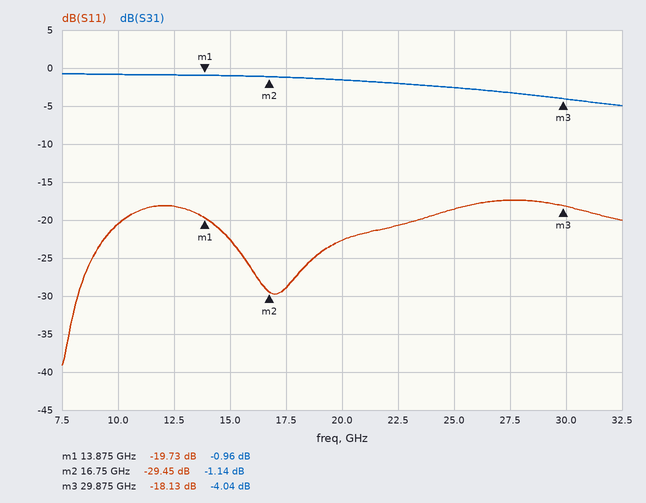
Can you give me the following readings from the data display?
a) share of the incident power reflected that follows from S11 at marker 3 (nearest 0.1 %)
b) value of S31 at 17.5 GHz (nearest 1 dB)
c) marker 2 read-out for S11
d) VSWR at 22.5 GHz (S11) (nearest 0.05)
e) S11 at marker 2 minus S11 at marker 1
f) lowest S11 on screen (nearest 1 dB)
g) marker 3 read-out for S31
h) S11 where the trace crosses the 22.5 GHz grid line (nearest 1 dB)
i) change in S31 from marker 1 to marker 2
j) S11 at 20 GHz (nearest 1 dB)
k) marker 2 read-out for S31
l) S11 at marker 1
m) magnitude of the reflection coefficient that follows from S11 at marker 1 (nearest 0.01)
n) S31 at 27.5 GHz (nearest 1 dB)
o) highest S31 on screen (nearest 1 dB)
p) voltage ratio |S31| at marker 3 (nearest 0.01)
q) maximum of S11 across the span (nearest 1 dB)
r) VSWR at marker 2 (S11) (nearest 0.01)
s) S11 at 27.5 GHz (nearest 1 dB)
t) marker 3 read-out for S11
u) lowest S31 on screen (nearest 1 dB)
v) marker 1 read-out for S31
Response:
1.5 %
-1 dB
-29.45 dB
1.20
-9.72 dB
-39 dB
-4.04 dB
-21 dB
-0.18 dB
-23 dB
-1.14 dB
-19.73 dB
0.10
-3 dB
-1 dB
0.63
-17 dB
1.07
-17 dB
-18.13 dB
-5 dB
-0.96 dB
